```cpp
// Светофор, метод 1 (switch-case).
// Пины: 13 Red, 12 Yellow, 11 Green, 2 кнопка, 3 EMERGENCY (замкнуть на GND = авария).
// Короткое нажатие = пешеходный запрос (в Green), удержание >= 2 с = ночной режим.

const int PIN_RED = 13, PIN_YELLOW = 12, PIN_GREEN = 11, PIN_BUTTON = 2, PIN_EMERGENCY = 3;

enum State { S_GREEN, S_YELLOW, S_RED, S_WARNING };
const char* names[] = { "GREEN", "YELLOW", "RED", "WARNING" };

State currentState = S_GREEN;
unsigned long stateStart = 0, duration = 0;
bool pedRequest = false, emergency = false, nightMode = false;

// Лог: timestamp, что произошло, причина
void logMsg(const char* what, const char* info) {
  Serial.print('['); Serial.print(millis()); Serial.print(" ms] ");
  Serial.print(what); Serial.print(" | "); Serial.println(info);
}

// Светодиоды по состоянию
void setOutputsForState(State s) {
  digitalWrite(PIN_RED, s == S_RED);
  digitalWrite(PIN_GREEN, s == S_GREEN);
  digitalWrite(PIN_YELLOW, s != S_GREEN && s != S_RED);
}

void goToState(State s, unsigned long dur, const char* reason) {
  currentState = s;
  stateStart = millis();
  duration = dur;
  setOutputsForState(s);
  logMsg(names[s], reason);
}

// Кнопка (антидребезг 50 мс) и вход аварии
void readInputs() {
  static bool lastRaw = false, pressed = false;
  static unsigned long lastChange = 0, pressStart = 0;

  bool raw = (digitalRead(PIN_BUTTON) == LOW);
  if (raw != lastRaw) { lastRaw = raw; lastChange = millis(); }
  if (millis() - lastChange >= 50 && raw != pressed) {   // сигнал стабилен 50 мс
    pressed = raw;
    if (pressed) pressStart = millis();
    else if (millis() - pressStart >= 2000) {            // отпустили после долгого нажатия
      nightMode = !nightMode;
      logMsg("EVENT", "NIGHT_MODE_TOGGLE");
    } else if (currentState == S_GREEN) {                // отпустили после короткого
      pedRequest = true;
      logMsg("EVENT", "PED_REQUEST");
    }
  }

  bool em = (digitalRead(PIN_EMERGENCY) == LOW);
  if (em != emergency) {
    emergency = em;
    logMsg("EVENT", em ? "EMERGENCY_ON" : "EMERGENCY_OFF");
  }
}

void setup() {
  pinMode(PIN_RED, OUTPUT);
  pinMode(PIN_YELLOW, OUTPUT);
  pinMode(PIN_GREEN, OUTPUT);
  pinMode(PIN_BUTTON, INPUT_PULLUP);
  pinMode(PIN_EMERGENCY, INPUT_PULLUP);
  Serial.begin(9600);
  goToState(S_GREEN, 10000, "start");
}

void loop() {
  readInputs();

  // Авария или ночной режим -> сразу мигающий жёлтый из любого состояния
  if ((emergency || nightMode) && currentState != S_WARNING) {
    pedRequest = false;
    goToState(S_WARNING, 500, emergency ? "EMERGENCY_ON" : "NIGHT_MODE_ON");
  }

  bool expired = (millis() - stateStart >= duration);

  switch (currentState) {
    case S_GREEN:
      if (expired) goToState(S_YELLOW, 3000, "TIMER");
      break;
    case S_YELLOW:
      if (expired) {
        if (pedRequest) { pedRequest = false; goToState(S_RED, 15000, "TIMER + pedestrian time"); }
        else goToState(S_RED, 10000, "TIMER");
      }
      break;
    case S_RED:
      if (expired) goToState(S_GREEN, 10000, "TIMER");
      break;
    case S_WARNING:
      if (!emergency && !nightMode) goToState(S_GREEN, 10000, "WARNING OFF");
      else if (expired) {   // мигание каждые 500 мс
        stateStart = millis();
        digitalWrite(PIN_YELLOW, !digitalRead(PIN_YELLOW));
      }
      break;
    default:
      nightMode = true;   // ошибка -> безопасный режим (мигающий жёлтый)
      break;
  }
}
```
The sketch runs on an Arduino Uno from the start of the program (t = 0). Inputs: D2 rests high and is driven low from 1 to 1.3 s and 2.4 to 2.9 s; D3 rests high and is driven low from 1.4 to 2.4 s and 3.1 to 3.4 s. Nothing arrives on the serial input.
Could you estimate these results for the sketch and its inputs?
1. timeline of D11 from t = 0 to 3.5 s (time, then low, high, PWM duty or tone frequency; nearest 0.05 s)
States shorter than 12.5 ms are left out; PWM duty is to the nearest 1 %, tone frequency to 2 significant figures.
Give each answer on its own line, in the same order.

0 s high; 1.4 s low; 2.4 s high; 3.1 s low; 3.4 s high
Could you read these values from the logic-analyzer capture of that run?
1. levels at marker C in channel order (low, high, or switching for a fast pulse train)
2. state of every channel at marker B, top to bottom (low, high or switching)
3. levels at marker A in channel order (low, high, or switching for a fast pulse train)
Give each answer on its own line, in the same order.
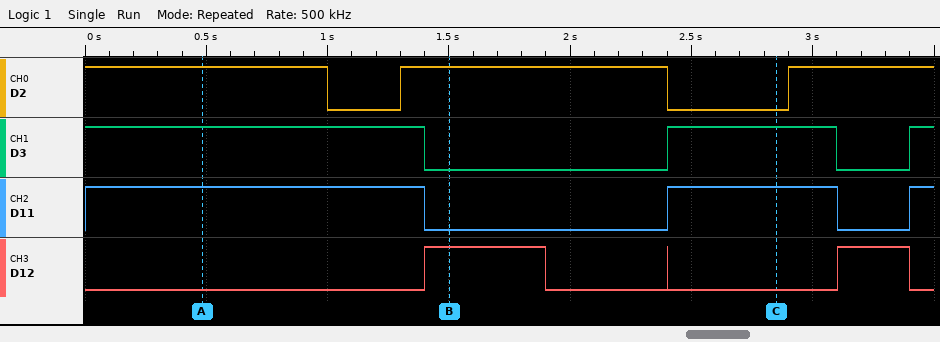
D2 low, D3 high, D11 high, D12 low
D2 high, D3 low, D11 low, D12 high
D2 high, D3 high, D11 high, D12 low
